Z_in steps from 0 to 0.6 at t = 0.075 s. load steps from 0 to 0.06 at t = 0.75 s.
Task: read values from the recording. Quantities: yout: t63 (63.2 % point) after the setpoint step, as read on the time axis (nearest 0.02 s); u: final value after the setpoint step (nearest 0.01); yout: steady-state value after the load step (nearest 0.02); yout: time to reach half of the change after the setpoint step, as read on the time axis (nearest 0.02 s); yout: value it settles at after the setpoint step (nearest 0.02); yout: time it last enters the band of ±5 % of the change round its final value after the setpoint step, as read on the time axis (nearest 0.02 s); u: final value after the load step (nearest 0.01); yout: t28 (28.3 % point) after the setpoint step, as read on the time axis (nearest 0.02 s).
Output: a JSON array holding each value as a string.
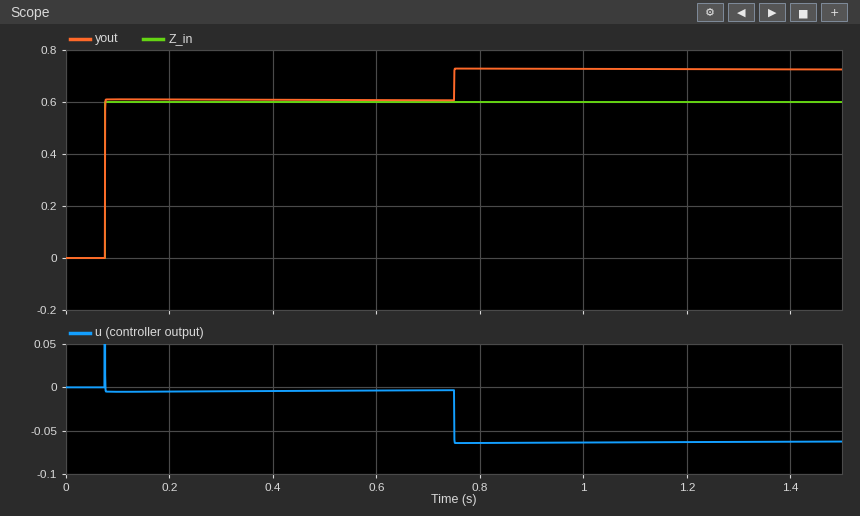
["0.08 s", "0.00", "0.72", "0.08 s", "0.60", "0.08 s", "-0.06", "0.08 s"]
